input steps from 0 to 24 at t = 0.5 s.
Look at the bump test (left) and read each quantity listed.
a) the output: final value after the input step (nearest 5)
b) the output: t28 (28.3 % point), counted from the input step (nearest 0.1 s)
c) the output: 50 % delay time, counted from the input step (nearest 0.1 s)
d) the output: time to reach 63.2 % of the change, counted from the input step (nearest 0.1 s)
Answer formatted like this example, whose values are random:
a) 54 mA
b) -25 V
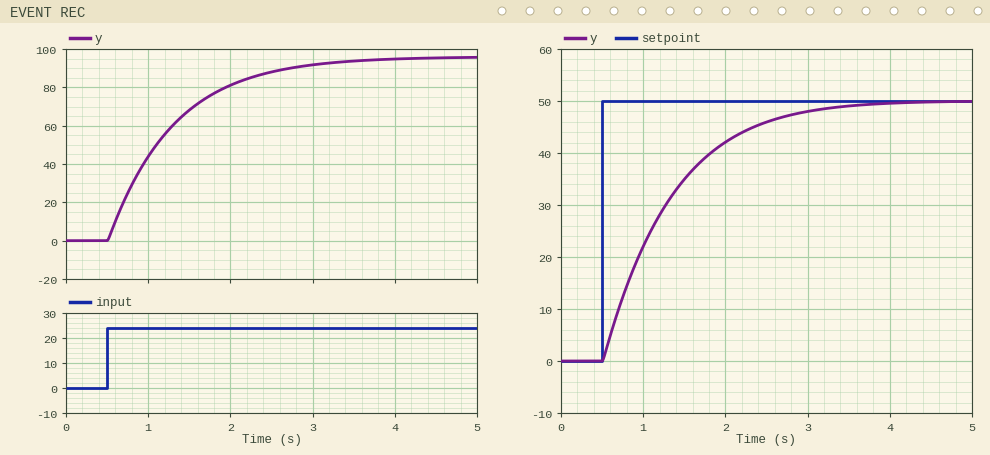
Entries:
a) 95
b) 0.3 s
c) 0.6 s
d) 0.8 s
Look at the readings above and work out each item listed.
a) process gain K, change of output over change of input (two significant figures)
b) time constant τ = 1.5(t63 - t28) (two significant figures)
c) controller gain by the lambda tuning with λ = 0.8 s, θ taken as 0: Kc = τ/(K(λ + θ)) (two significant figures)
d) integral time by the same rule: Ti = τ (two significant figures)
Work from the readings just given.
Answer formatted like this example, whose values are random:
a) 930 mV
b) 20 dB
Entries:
a) 4.0
b) 0.75 s
c) 0.23
d) 0.75 s
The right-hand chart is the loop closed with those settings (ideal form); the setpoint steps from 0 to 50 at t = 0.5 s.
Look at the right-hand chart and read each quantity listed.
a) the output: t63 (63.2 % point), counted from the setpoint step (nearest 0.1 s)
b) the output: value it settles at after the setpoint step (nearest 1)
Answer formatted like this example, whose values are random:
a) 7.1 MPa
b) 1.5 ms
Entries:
a) 0.8 s
b) 50
